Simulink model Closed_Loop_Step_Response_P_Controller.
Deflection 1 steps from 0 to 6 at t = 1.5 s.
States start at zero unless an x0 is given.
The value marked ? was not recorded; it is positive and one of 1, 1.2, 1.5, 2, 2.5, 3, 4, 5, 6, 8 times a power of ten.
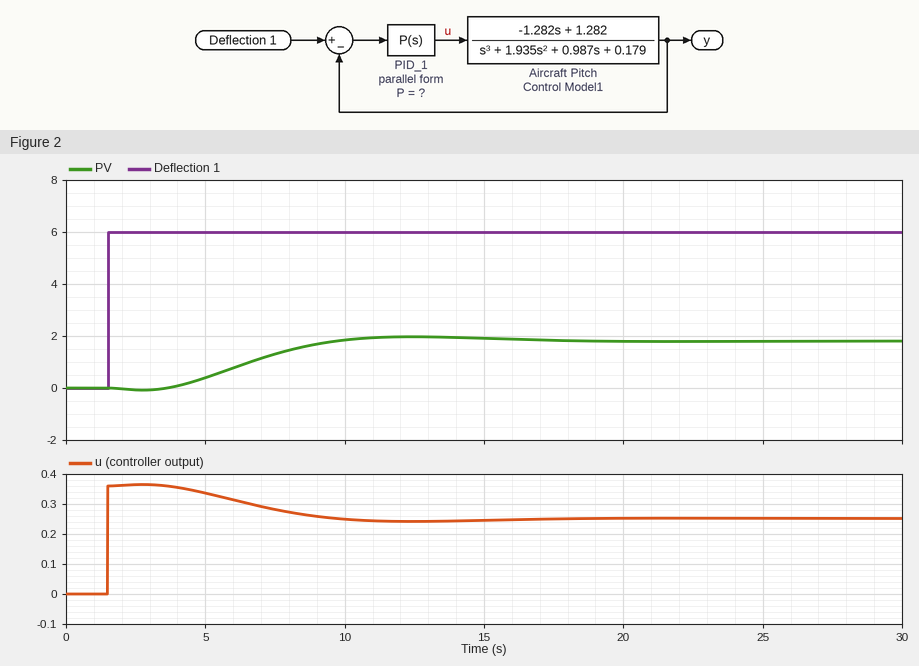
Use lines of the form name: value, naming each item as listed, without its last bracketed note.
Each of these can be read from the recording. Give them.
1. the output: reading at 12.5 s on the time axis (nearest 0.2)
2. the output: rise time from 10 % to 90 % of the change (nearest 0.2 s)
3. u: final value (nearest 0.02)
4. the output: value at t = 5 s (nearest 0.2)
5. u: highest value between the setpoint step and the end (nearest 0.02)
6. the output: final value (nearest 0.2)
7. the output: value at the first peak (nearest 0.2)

the output: reading at 12.5 s on the time axis: 2.0
the output: rise time from 10 % to 90 % of the change: 4.4 s
u: final value: 0.26
the output: value at t = 5 s: 0.4
u: highest value between the setpoint step and the end: 0.36
the output: final value: 1.8
the output: value at the first peak: 2.0
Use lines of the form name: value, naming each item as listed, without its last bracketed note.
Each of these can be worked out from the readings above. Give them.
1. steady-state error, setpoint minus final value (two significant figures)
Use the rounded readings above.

steady-state error, setpoint minus final value: 4.2
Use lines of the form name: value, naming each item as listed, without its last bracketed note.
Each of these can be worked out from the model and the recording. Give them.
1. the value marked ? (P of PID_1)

the value marked ?: 0.06
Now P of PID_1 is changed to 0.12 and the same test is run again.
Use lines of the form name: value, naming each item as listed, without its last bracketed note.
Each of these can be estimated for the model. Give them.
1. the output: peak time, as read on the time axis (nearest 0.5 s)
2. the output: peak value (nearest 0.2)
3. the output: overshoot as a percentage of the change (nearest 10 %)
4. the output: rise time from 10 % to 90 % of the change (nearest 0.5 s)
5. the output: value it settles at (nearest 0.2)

the output: peak time, as read on the time axis: 10.5 s
the output: peak value: 3.4
the output: overshoot as a percentage of the change: 20 %
the output: rise time from 10 % to 90 % of the change: 3.0 s
the output: value it settles at: 2.8
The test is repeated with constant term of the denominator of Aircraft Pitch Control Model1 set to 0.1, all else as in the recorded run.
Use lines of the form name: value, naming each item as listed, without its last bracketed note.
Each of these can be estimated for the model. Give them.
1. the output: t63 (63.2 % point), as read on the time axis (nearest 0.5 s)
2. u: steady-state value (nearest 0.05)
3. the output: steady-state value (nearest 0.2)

the output: t63 (63.2 % point), as read on the time axis: 8.5 s
u: steady-state value: 0.20
the output: steady-state value: 2.6
